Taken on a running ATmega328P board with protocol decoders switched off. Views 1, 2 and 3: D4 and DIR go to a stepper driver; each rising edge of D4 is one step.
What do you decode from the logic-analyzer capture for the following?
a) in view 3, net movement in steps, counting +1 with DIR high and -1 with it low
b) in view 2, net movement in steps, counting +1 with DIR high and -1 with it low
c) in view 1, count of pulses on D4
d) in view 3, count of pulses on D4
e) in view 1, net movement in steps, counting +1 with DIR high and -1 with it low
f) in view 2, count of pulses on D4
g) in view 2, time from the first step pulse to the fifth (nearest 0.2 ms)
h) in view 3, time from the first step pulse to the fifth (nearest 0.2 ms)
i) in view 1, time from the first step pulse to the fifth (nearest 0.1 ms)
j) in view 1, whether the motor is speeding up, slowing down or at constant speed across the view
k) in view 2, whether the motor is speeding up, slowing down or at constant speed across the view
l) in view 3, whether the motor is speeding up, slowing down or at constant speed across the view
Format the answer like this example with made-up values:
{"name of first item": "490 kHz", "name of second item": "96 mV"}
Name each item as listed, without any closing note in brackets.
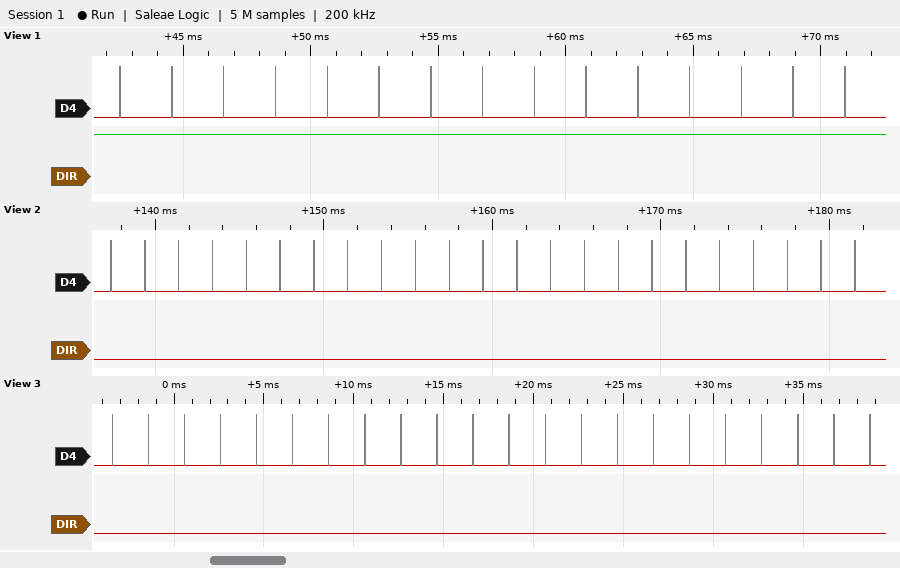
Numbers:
{"in view 3, net movement in steps, counting +1 with DIR high and -1 with it low": "-22", "in view 2, net movement in steps, counting +1 with DIR high and -1 with it low": "-23", "in view 1, count of pulses on D4": "15", "in view 3, count of pulses on D4": "22", "in view 1, net movement in steps, counting +1 with DIR high and -1 with it low": "+15", "in view 2, count of pulses on D4": "23", "in view 2, time from the first step pulse to the fifth": "8.0 ms", "in view 3, time from the first step pulse to the fifth": "8.0 ms", "in view 1, time from the first step pulse to the fifth": "8.1 ms", "in view 1, whether the motor is speeding up, slowing down or at constant speed across the view": "constant speed", "in view 2, whether the motor is speeding up, slowing down or at constant speed across the view": "constant speed", "in view 3, whether the motor is speeding up, slowing down or at constant speed across the view": "constant speed"}
